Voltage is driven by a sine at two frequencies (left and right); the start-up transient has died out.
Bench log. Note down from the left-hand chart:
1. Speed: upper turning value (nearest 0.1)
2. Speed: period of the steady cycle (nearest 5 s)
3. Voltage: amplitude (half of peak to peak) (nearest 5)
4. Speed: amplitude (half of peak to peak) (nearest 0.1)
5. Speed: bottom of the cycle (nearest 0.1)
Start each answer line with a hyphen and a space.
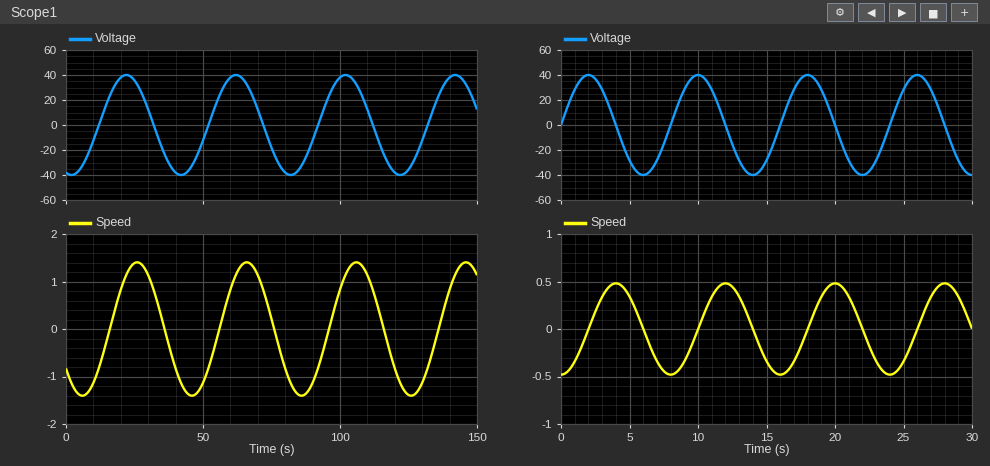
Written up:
- 1.4
- 40 s
- 40
- 1.4
- -1.4
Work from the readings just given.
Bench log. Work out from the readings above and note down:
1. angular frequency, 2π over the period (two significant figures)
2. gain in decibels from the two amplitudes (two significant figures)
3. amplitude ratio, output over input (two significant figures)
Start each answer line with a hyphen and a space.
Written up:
- 0.16 rad/s
- -29 dB
- 0.035
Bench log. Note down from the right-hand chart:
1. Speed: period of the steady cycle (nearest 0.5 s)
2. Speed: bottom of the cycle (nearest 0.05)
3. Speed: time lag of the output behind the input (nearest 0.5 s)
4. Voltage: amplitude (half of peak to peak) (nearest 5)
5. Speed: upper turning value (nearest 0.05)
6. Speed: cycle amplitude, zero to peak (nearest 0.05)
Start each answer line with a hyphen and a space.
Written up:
- 8.0 s
- -0.50
- 2.0 s
- 40
- 0.50
- 0.50
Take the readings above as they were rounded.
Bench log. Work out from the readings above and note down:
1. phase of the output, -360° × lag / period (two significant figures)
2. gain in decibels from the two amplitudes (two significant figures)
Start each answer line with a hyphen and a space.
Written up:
- -90°
- -38 dB
